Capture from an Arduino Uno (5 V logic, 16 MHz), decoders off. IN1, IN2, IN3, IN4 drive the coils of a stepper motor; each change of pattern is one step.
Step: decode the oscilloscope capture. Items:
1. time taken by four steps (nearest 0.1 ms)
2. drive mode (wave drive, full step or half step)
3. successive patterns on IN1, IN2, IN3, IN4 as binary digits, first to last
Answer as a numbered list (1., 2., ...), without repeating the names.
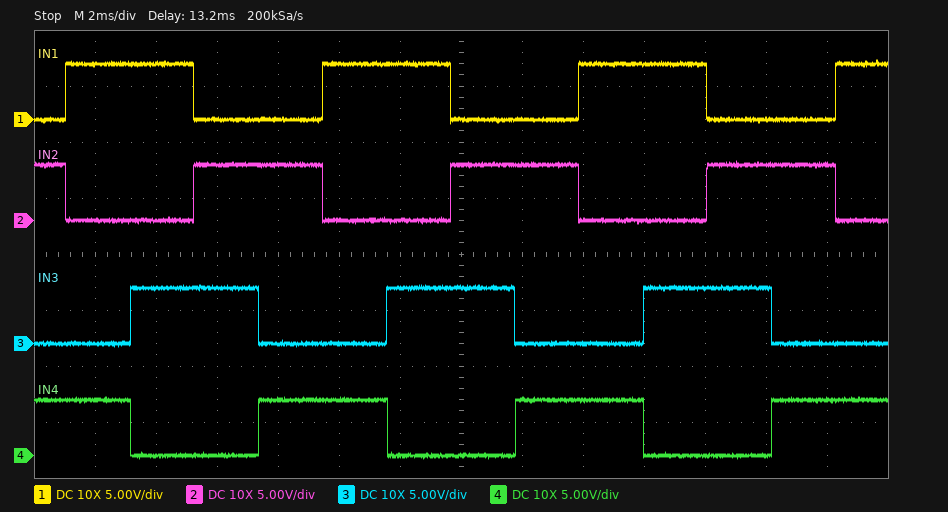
1. 8.4 ms
2. full step
3. 0101 1001 1010 0110 0101 1001 1010 0110 0101 1001 1010 0110 0101 1001
